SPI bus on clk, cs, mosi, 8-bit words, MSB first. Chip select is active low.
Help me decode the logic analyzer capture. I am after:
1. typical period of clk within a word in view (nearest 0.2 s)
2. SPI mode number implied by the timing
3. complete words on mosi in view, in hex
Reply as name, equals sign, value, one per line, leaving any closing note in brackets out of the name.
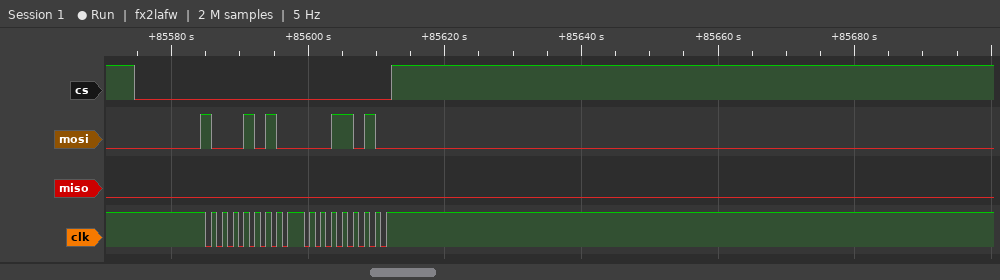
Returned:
typical period of clk within a word in view = 1.6 s
SPI mode number implied by the timing = 2
complete words on mosi in view, in hex = 8A, 1A
